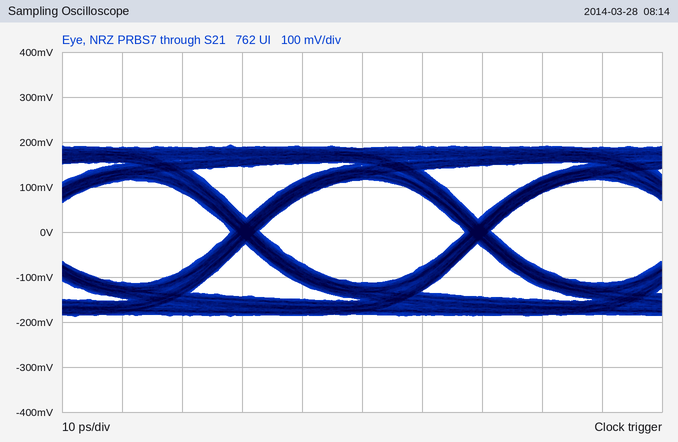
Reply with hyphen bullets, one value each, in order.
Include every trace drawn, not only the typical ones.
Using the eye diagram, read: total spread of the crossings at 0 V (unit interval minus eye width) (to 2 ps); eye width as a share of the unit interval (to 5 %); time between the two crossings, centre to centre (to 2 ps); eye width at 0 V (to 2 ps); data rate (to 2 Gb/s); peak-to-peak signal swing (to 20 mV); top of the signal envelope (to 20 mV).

- 4 ps
- 90 %
- 38 ps
- 34 ps
- 26 Gb/s
- 380 mV
- 200 mV
